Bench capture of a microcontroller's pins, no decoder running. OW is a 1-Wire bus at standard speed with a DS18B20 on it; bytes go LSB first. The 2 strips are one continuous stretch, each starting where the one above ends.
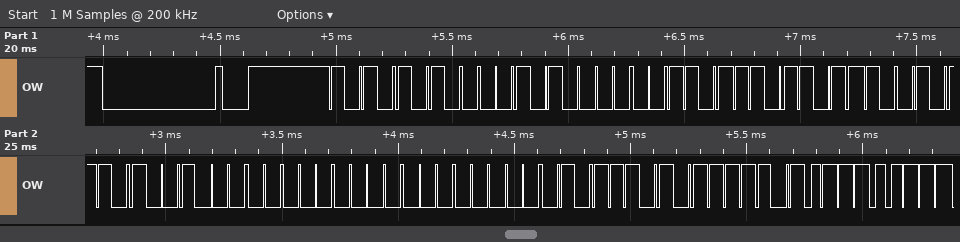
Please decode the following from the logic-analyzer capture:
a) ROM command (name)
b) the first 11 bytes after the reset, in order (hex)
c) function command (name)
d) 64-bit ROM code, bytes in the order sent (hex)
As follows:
Match ROM
55 28 B0 DB 69 09 00 00 BA BE CE
Read Scratchpad
28 B0 DB 69 09 00 00 BA
